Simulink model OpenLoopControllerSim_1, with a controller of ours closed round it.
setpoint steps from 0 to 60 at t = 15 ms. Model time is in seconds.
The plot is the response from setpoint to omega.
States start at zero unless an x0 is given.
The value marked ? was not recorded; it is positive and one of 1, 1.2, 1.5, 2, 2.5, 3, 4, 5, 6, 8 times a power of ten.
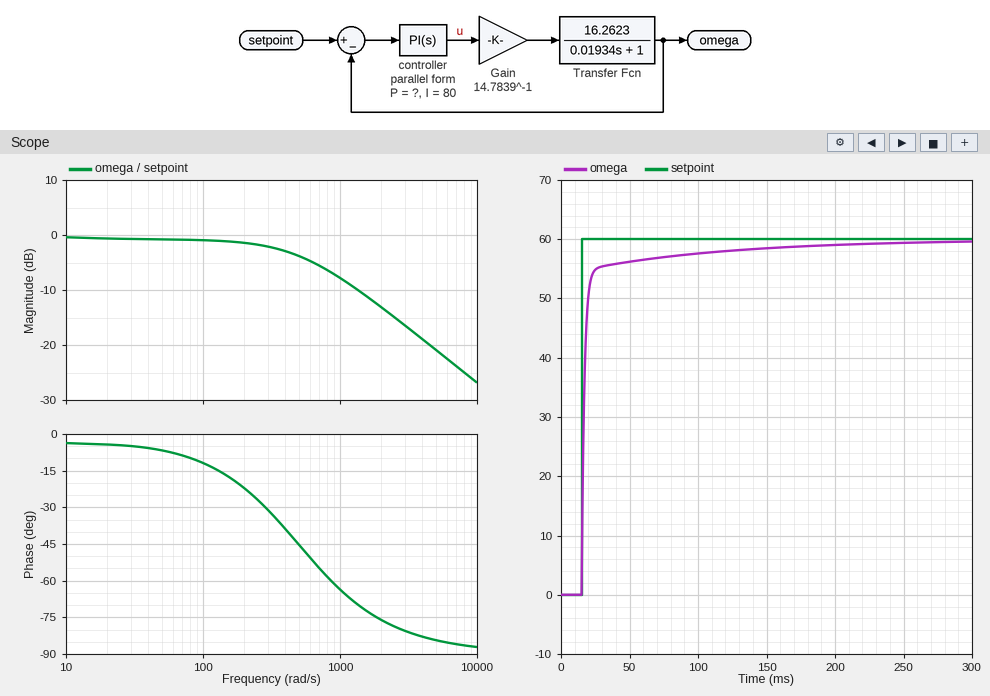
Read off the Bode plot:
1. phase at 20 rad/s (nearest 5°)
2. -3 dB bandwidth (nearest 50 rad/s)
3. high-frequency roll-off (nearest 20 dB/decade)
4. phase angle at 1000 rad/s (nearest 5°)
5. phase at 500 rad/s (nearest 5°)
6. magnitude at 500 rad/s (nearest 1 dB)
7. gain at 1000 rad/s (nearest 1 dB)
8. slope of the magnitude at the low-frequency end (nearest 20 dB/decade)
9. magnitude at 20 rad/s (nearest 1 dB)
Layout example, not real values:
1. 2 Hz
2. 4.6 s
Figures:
1. -5°
2. 450 rad/s
3. -20 dB/decade
4. -65°
5. -45°
6. -4 dB
7. -8 dB
8. 0 dB/decade
9. -1 dB
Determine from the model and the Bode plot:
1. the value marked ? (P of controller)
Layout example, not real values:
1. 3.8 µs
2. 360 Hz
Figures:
1. 8
